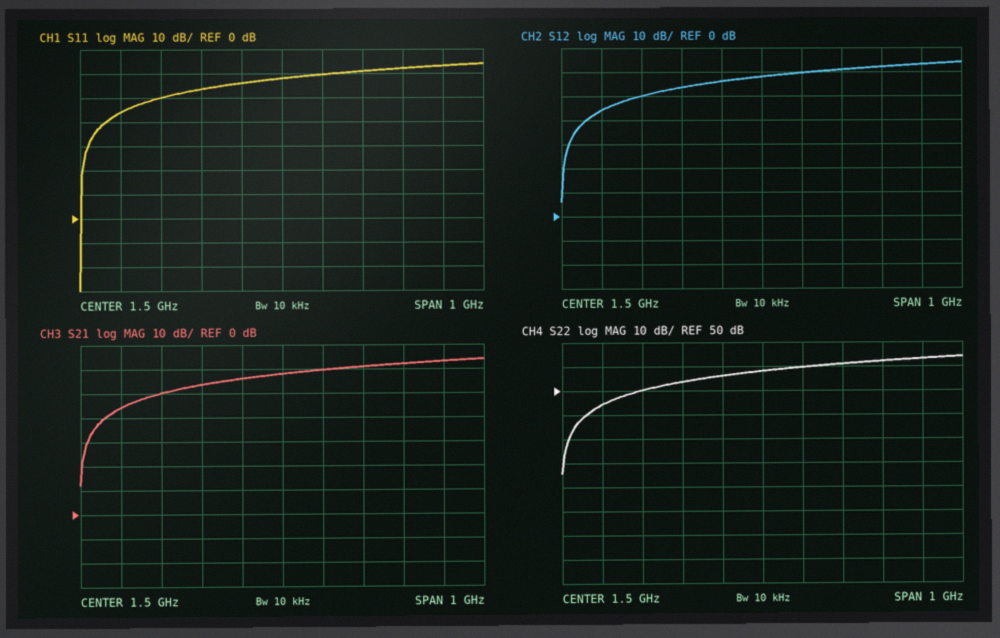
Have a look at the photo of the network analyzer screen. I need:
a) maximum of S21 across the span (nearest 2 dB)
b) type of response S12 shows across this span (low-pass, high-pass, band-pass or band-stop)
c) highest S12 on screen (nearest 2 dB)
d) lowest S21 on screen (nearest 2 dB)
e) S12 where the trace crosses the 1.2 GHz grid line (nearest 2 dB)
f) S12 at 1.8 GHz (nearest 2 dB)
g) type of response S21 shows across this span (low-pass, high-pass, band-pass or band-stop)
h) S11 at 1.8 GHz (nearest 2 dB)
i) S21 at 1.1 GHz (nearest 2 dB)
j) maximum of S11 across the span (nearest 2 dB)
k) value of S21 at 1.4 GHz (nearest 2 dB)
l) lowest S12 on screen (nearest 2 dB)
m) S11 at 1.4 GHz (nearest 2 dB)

64 dB
high-pass
64 dB
12 dB
50 dB
62 dB
high-pass
62 dB
44 dB
64 dB
56 dB
6 dB
56 dB
